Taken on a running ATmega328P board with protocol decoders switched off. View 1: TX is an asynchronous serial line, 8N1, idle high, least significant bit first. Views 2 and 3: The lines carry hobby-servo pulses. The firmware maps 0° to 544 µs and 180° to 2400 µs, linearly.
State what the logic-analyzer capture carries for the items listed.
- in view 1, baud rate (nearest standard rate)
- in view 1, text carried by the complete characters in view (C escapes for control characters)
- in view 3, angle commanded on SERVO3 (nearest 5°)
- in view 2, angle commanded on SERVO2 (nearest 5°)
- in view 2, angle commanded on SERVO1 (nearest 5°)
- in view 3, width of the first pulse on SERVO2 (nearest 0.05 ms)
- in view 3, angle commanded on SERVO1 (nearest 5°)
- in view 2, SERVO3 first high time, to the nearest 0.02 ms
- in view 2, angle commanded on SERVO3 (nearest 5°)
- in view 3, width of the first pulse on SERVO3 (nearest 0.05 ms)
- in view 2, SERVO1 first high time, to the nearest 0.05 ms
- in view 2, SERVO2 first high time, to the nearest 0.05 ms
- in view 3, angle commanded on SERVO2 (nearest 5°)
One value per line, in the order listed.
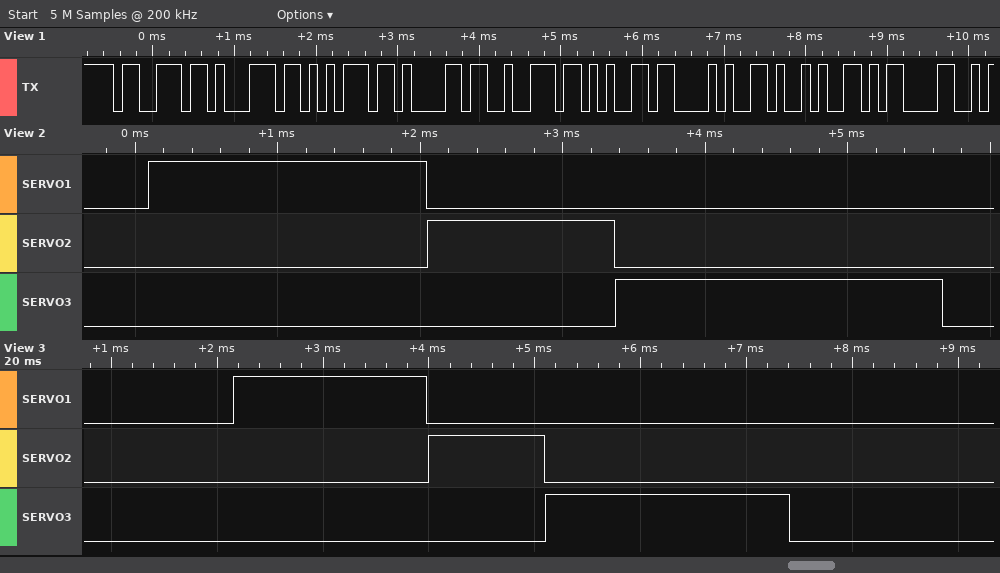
9600 baud
"square()\r"
170°
75°
135°
1.10 ms
125°
2.30 ms
170°
2.30 ms
1.95 ms
1.30 ms
55°
